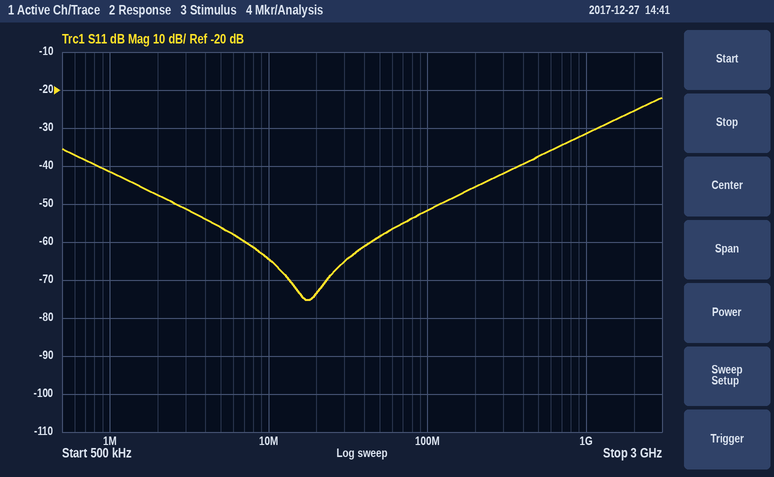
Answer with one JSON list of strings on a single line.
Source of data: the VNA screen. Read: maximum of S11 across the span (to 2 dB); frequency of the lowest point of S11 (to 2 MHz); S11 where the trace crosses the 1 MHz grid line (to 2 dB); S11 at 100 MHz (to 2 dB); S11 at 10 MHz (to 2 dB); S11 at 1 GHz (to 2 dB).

["-22 dB", "18 MHz", "-42 dB", "-52 dB", "-64 dB", "-32 dB"]
